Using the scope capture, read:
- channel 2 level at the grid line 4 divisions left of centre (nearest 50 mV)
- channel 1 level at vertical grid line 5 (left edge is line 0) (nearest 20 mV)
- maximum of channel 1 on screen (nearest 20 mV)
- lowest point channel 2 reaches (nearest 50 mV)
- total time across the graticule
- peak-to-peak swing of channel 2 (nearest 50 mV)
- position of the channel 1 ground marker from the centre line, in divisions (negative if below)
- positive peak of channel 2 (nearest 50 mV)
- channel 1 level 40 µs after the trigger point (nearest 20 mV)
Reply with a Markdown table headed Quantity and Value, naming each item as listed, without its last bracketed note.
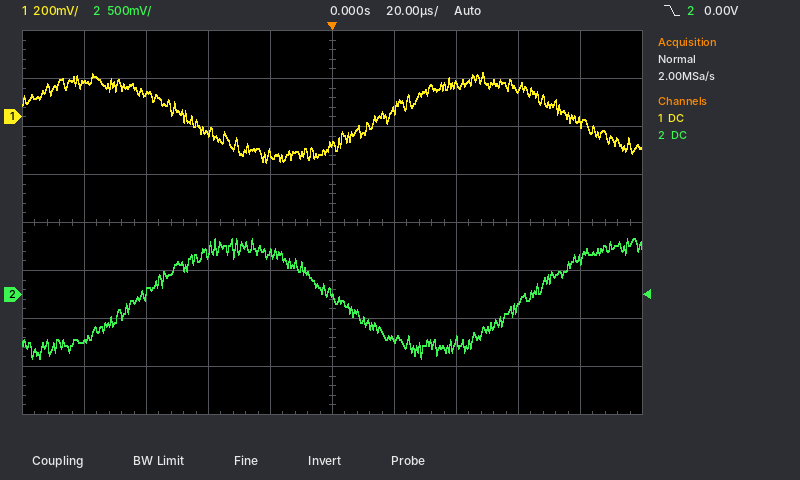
| Quantity | Value |
|---|---|
| channel 2 level at the grid line 4 divisions left of centre | -500 mV |
| channel 1 level at vertical grid line 5 (left edge is line 0) | -120 mV |
| maximum of channel 1 on screen | 180 mV |
| lowest point channel 2 reaches | -650 mV |
| total time across the graticule | 200 µs |
| peak-to-peak swing of channel 2 | 1.25 V |
| position of the channel 1 ground marker from the centre line, in divisions | +2.2 div |
| positive peak of channel 2 | 600 mV |
| channel 1 level 40 µs after the trigger point | 140 mV |
